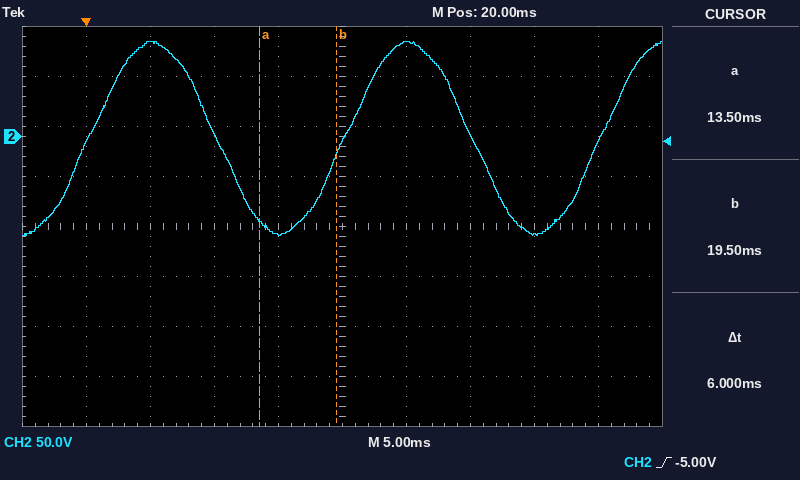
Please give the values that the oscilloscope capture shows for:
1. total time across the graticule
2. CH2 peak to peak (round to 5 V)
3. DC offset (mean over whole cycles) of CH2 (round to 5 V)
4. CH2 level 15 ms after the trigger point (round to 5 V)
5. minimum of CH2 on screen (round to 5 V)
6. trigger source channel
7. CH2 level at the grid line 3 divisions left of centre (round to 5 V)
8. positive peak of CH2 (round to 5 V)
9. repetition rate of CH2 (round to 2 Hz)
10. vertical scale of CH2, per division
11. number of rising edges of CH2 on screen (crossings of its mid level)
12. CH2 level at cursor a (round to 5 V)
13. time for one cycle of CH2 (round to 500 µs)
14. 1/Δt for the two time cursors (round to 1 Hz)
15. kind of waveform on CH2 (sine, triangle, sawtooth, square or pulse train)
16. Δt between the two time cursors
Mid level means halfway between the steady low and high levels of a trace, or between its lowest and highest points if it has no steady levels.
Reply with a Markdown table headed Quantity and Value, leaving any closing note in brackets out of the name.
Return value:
| Quantity | Value |
|---|---|
| total time across the graticule | 50 ms |
| CH2 peak to peak | 195 V |
| DC offset (mean over whole cycles) of CH2 | 0 V |
| CH2 level 15 ms after the trigger point | -100 V |
| minimum of CH2 on screen | -100 V |
| trigger source channel | CH2 |
| CH2 level at the grid line 3 divisions left of centre | 95 V |
| positive peak of CH2 | 95 V |
| repetition rate of CH2 | 50 Hz |
| vertical scale of CH2, per division | 50 V |
| number of rising edges of CH2 on screen | 3 |
| CH2 level at cursor a | -85 V |
| time for one cycle of CH2 | 20.0 ms |
| 1/Δt for the two time cursors | 167 Hz |
| kind of waveform on CH2 | sine |
| Δt between the two time cursors | 6 ms |
